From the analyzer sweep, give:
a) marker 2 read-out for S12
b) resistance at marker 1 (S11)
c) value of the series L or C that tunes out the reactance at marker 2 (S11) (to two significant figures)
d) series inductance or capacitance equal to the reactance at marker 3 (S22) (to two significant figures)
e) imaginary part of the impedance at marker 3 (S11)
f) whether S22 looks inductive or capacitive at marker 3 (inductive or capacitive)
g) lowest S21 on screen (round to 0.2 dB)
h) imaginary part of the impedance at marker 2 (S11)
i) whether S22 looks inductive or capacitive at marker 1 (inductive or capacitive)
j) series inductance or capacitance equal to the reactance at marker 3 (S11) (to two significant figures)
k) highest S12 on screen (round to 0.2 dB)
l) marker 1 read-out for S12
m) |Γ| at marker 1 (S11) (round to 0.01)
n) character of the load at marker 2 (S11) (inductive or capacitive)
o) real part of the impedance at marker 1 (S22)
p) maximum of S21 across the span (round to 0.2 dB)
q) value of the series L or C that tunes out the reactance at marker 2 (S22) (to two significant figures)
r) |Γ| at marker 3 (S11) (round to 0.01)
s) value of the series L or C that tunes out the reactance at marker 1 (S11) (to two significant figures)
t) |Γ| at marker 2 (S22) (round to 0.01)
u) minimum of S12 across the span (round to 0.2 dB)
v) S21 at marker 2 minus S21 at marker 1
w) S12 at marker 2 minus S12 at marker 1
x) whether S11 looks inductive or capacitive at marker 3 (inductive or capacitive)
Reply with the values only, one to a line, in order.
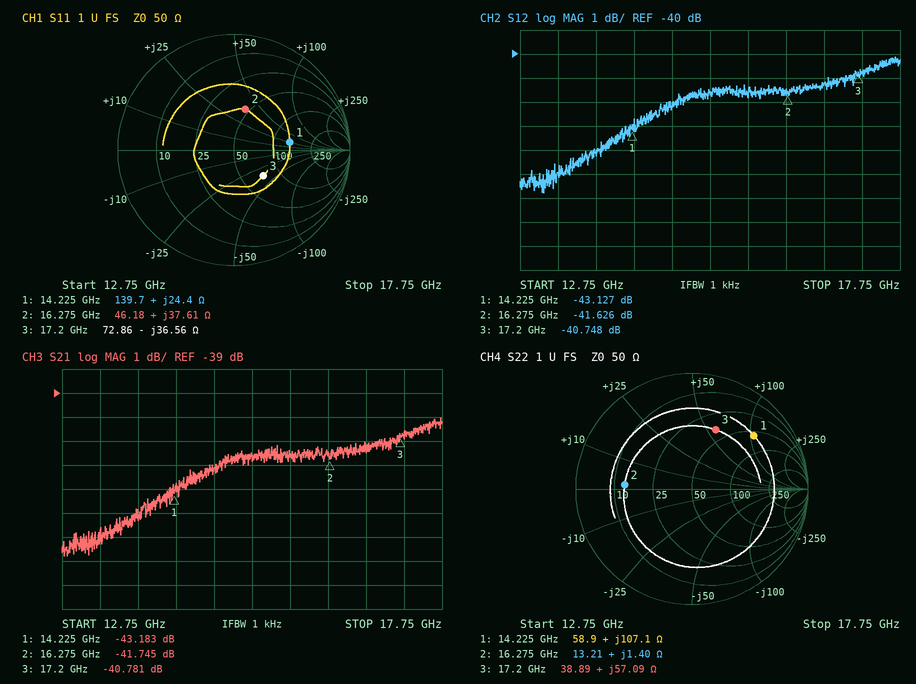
-41.626 dB
139.7 Ω
260 fF
530 pH
-36.56 Ω
inductive
-45.8 dB
+37.61 Ω
inductive
250 fF
-40.2 dB
-43.127 dB
0.49
inductive
58.9 Ω
-40.0 dB
7.0 pF
0.34
460 fF
0.58
-45.8 dB
1.438 dB
1.501 dB
capacitive
